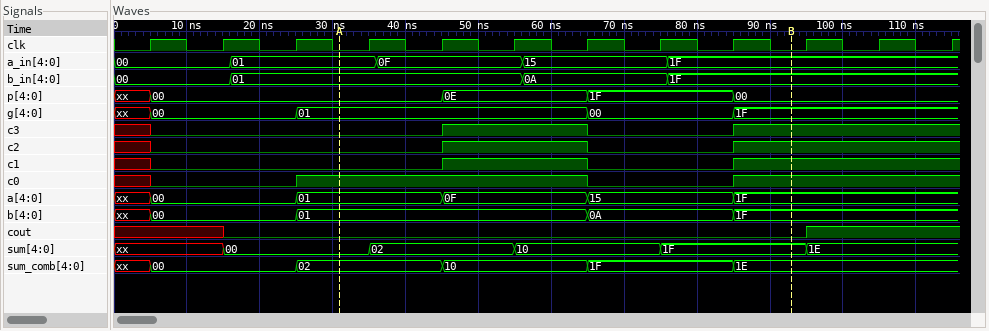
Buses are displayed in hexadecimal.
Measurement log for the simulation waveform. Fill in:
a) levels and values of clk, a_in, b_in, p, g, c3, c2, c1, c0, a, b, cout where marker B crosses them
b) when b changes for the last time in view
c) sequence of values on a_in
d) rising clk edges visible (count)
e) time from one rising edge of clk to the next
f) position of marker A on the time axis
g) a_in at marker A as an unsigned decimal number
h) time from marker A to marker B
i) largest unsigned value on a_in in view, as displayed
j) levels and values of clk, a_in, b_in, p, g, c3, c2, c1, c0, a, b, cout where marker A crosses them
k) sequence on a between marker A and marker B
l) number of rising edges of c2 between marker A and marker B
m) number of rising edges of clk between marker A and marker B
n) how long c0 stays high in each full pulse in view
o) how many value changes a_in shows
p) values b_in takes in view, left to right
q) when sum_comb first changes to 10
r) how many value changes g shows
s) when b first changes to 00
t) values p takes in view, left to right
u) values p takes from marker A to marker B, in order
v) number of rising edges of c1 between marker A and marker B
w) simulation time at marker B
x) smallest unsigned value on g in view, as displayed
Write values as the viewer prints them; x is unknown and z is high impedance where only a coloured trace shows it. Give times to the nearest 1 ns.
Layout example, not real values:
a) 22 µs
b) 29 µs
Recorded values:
a) clk=0, a_in=1F, b_in=1F, p=00, g=1F, c3=1, c2=1, c1=1, c0=1, a=1F, b=1F, cout=0
b) 85 ns
c) 00, 01, 0F, 15, 1F
d) 12
e) 10 ns
f) 31 ns
g) 1
h) 62 ns
i) 1F
j) clk=0, a_in=01, b_in=01, p=00, g=01, c3=0, c2=0, c1=0, c0=1, a=01, b=01, cout=0
k) 01, 0F, 15, 1F
l) 2
m) 6
n) 40 ns
o) 4
p) 00, 01, 0A, 1F
q) 45 ns
r) 4
s) 5 ns
t) xx, 00, 0E, 1F, 00
u) 00, 0E, 1F, 00
v) 2
w) 93 ns
x) 00
